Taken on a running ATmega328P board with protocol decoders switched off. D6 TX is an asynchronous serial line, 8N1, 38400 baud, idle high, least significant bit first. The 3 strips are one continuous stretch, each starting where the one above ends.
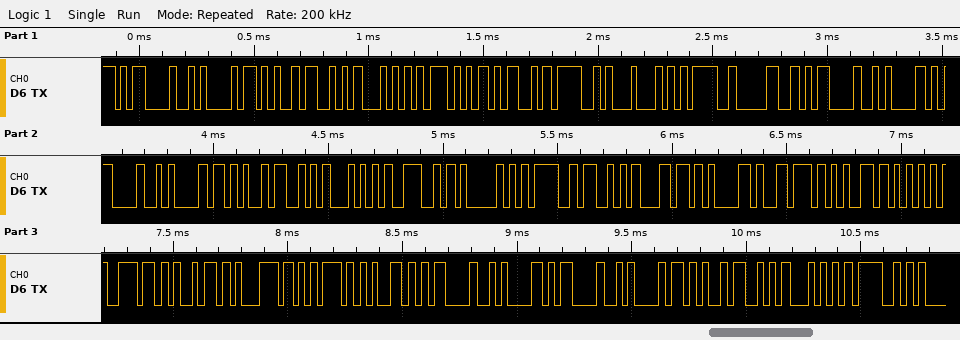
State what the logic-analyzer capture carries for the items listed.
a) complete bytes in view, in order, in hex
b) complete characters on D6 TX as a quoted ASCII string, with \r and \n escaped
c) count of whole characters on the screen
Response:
0D 0A 2B 53 54 57 4D 4F 44 3D 30 0D 0A 0D 0A 2B 53 54 4E 41 3D 53 6C 61 76 65 55 6E 69 71 75 65 0D 0A 0D 0A 2B 53 54 4F
"\r\n+STWMOD=0\r\n\r\n+STNA=SlaveUnique\r\n\r\n+STO"
40
